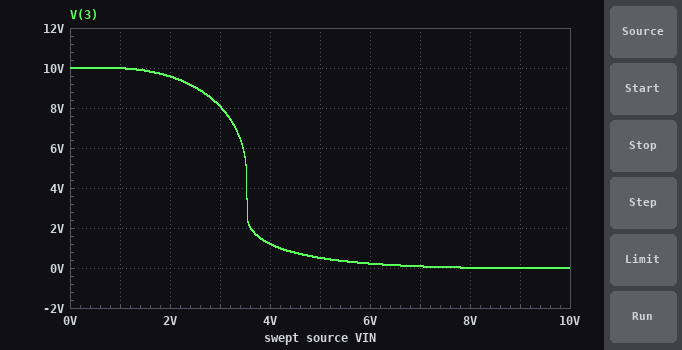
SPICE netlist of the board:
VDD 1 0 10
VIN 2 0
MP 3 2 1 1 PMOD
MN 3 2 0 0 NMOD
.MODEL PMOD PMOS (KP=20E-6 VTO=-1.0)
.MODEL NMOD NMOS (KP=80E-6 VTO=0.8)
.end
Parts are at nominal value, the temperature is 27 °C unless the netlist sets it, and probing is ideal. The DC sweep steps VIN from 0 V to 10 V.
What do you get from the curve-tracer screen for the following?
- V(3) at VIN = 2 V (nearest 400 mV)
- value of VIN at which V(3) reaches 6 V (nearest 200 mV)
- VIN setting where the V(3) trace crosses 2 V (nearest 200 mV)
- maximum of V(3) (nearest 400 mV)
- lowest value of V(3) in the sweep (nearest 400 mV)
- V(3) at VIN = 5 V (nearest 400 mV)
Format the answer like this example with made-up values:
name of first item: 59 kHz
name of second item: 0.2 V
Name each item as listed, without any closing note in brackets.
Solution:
V(3) at VIN = 2 V: 9.6 V
value of VIN at which V(3) reaches 6 V: 3.4 V
VIN setting where the V(3) trace crosses 2 V: 3.6 V
maximum of V(3): 10.0 V
lowest value of V(3) in the sweep: 0 V
V(3) at VIN = 5 V: 400 mV
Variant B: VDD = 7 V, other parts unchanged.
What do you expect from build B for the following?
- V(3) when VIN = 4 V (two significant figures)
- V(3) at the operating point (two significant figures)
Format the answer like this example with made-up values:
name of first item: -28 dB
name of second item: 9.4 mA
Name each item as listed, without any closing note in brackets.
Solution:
V(3) when VIN = 4 V: 160 mV
V(3) at the operating point: 7.0 V
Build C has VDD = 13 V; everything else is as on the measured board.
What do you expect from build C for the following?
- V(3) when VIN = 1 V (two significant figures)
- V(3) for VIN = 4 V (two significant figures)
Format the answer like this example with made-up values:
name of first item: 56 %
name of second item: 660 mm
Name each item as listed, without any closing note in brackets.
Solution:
V(3) when VIN = 1 V: 13 V
V(3) for VIN = 4 V: 9.8 V
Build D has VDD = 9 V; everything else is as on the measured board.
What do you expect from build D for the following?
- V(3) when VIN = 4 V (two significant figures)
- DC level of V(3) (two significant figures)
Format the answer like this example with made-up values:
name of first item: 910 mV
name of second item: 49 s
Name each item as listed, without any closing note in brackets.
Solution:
V(3) when VIN = 4 V: 700 mV
DC level of V(3): 9.0 V
